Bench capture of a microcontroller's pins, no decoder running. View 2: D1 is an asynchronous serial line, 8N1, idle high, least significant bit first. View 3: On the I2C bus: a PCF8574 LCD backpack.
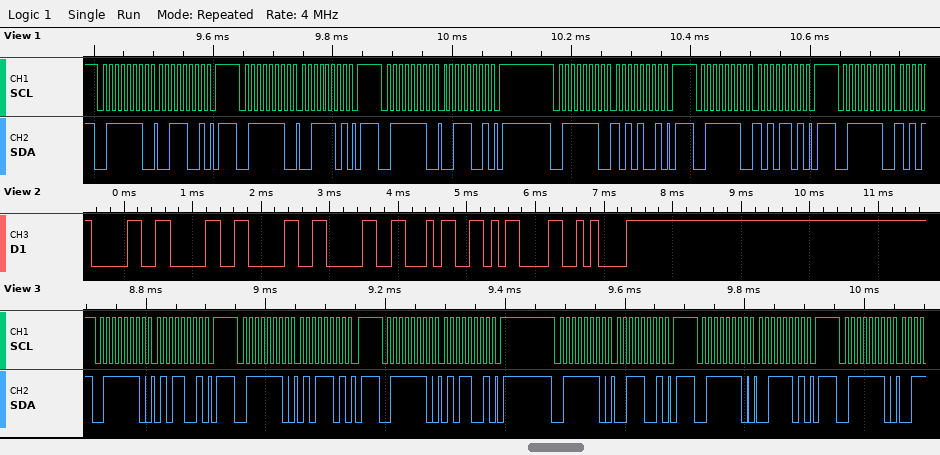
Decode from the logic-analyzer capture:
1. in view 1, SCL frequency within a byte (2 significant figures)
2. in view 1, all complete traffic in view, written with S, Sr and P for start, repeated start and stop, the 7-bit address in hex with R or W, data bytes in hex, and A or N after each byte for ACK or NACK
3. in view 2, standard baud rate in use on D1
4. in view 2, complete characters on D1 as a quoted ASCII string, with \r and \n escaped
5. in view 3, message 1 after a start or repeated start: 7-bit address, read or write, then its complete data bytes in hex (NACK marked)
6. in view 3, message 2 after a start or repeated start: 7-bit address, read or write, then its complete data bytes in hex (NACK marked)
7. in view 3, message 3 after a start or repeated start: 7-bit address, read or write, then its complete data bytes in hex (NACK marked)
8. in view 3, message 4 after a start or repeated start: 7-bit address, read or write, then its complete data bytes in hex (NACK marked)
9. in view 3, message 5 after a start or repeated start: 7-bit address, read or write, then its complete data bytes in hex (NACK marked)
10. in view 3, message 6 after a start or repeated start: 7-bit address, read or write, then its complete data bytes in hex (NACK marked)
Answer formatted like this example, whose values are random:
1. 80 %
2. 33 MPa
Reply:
1. 100 kHz
2. S 3FW A 39 A P S 3FW A 3D A P S 3FW A 39 A P S 3FW A A9 A P S 3FW A AD A P S 3FW A
3. 9600 baud
4. "00004\r\n"
5. 0x3F write: 59
6. 0x3F write: 5D
7. 0x3F write: 59
8. 0x3F write: 39
9. 0x3F write: 3D
10. 0x3F write
